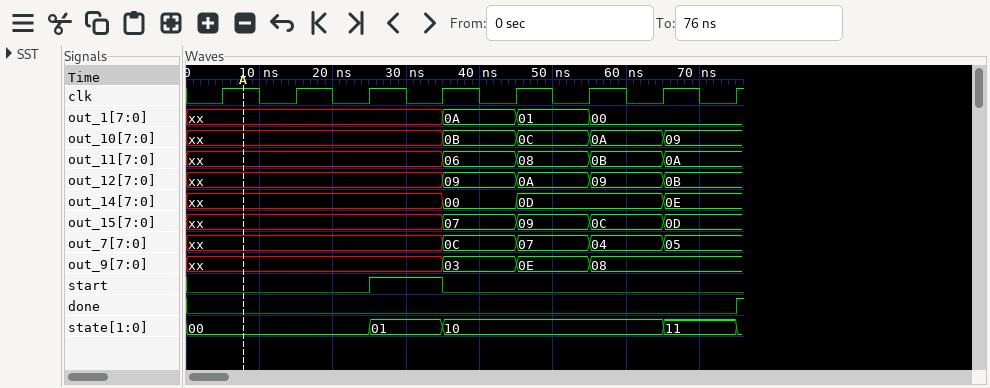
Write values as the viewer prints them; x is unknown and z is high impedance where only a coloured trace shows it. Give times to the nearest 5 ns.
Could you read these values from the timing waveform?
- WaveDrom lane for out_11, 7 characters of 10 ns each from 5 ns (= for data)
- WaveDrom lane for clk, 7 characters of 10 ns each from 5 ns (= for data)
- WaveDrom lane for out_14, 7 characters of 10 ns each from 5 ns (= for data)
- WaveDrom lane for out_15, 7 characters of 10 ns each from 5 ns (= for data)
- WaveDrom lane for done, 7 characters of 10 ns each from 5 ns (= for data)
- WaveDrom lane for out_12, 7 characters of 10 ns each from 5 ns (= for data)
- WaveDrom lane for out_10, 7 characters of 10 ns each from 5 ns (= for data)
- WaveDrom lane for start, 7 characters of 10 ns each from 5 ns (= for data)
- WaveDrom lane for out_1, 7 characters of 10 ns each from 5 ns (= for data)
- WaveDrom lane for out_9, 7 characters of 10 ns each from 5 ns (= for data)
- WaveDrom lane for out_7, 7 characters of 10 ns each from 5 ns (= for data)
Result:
{name: 'out_11', wave: 'x..====', data: '06 08 0B 0A'}
{name: 'clk', wave: 'p......'}
{name: 'out_14', wave: 'x..==.=', data: '00 0D 0E'}
{name: 'out_15', wave: 'x..====', data: '07 09 0C 0D'}
{name: 'done', wave: '0......'}
{name: 'out_12', wave: 'x..====', data: '09 0A 09 0B'}
{name: 'out_10', wave: 'x..====', data: '0B 0C 0A 09'}
{name: 'start', wave: '0.10...'}
{name: 'out_1', wave: 'x..===.', data: '0A 01 00'}
{name: 'out_9', wave: 'x..===.', data: '03 0E 08'}
{name: 'out_7', wave: 'x..====', data: '0C 07 04 05'}
